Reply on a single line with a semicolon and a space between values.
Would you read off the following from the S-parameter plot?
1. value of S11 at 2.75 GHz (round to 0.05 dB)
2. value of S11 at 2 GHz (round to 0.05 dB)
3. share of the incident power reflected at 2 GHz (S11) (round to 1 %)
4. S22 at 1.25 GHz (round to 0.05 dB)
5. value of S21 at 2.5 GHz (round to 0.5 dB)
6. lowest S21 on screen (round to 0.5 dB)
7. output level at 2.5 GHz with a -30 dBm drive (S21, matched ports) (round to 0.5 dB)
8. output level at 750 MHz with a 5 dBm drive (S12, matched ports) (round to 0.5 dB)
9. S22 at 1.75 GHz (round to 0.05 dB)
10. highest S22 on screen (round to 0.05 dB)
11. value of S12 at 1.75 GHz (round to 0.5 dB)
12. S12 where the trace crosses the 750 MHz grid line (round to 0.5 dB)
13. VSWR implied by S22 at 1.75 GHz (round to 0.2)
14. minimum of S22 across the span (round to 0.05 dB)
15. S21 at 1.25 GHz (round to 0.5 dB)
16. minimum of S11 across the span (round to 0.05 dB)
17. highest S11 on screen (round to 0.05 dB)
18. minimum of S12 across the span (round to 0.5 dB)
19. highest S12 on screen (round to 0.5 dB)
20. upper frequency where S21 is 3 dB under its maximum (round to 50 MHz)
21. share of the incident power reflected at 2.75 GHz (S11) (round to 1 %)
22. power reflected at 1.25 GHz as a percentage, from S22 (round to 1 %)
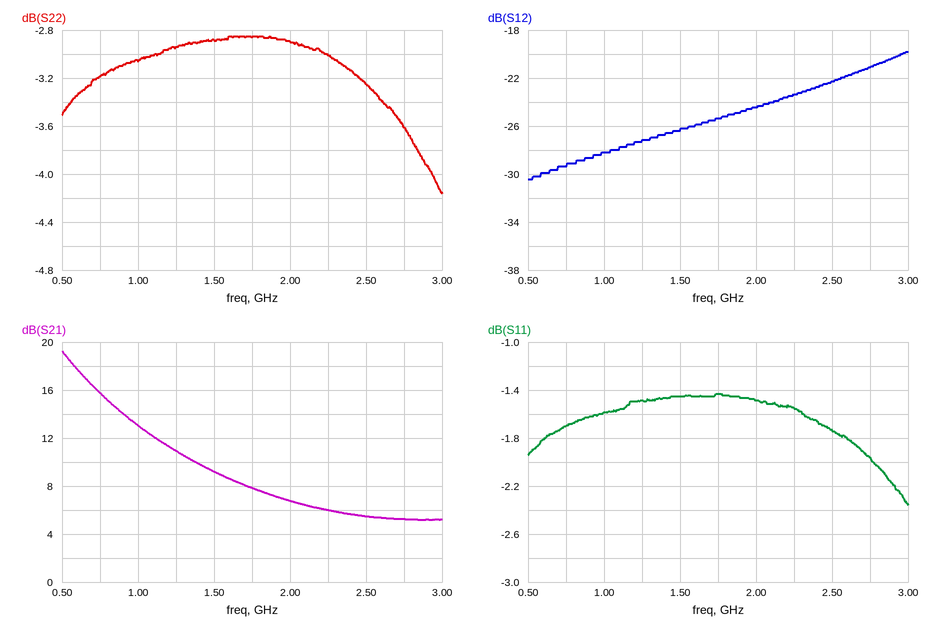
-1.95 dB; -1.50 dB; 71 %; -2.95 dB; 5.5 dB; 5.0 dB; -24.5 dBm; -24.5 dBm; -2.85 dB; -2.85 dB; -25.5 dB; -29.5 dB; 6.2; -4.15 dB; 11.0 dB; -2.35 dB; -1.45 dB; -30.5 dB; -20.0 dB; 700 MHz; 64 %; 51 %
